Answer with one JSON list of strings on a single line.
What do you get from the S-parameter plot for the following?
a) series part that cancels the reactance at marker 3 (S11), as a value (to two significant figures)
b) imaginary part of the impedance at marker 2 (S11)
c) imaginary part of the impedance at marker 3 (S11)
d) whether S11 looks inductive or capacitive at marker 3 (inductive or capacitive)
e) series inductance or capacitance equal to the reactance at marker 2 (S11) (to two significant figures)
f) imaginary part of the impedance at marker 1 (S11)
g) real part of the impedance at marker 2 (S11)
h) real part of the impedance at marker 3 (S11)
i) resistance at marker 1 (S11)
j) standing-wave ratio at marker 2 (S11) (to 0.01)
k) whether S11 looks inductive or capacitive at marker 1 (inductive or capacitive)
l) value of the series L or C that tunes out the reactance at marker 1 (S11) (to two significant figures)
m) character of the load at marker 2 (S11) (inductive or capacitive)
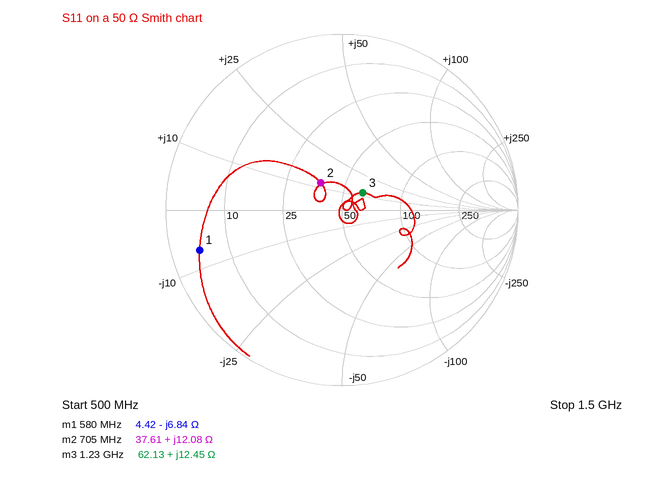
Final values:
["10 pF", "+12.08 Ω", "+12.45 Ω", "inductive", "2.7 nH", "-6.84 Ω", "37.61 Ω", "62.13 Ω", "4.42 Ω", "1.49", "capacitive", "1.9 nH", "inductive"]
